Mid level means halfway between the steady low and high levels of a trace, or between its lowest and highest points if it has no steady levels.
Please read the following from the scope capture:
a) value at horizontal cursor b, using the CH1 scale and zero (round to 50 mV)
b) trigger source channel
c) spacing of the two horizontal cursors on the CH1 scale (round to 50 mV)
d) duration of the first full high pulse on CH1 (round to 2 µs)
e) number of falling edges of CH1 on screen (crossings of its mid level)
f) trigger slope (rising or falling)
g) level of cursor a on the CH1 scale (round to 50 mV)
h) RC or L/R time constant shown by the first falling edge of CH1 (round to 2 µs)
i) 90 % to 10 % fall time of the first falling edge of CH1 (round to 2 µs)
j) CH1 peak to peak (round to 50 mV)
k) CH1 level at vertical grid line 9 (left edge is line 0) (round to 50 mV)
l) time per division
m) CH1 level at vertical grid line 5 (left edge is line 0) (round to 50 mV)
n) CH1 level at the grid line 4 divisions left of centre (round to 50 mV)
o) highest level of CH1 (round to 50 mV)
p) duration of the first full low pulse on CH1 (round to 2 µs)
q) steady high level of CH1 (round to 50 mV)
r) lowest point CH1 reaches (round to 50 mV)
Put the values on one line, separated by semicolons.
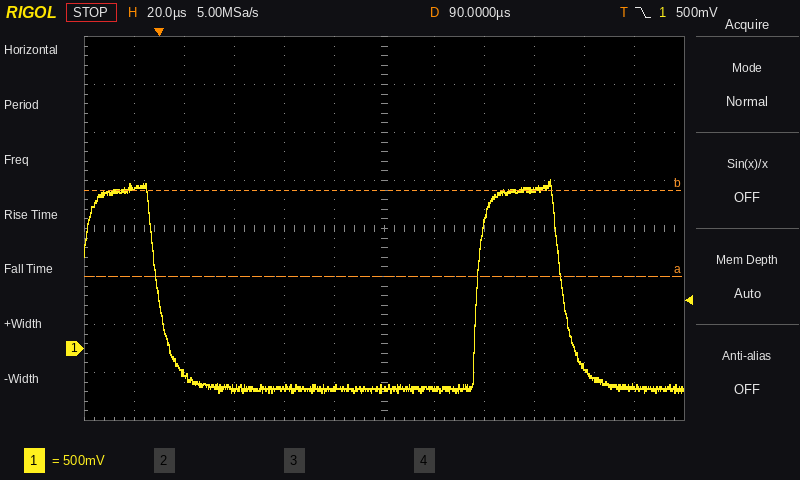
1.65 V; CH1; 900 mV; 34 µs; 2; falling; 750 mV; 6 µs; 12 µs; 2.20 V; 1.65 V; 20 µs; -400 mV; -250 mV; 1.75 V; 128 µs; 1.65 V; -450 mV
